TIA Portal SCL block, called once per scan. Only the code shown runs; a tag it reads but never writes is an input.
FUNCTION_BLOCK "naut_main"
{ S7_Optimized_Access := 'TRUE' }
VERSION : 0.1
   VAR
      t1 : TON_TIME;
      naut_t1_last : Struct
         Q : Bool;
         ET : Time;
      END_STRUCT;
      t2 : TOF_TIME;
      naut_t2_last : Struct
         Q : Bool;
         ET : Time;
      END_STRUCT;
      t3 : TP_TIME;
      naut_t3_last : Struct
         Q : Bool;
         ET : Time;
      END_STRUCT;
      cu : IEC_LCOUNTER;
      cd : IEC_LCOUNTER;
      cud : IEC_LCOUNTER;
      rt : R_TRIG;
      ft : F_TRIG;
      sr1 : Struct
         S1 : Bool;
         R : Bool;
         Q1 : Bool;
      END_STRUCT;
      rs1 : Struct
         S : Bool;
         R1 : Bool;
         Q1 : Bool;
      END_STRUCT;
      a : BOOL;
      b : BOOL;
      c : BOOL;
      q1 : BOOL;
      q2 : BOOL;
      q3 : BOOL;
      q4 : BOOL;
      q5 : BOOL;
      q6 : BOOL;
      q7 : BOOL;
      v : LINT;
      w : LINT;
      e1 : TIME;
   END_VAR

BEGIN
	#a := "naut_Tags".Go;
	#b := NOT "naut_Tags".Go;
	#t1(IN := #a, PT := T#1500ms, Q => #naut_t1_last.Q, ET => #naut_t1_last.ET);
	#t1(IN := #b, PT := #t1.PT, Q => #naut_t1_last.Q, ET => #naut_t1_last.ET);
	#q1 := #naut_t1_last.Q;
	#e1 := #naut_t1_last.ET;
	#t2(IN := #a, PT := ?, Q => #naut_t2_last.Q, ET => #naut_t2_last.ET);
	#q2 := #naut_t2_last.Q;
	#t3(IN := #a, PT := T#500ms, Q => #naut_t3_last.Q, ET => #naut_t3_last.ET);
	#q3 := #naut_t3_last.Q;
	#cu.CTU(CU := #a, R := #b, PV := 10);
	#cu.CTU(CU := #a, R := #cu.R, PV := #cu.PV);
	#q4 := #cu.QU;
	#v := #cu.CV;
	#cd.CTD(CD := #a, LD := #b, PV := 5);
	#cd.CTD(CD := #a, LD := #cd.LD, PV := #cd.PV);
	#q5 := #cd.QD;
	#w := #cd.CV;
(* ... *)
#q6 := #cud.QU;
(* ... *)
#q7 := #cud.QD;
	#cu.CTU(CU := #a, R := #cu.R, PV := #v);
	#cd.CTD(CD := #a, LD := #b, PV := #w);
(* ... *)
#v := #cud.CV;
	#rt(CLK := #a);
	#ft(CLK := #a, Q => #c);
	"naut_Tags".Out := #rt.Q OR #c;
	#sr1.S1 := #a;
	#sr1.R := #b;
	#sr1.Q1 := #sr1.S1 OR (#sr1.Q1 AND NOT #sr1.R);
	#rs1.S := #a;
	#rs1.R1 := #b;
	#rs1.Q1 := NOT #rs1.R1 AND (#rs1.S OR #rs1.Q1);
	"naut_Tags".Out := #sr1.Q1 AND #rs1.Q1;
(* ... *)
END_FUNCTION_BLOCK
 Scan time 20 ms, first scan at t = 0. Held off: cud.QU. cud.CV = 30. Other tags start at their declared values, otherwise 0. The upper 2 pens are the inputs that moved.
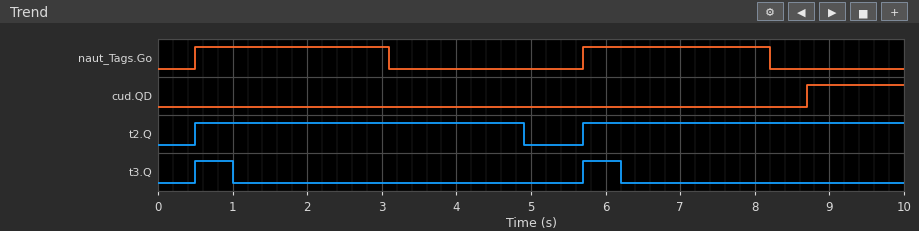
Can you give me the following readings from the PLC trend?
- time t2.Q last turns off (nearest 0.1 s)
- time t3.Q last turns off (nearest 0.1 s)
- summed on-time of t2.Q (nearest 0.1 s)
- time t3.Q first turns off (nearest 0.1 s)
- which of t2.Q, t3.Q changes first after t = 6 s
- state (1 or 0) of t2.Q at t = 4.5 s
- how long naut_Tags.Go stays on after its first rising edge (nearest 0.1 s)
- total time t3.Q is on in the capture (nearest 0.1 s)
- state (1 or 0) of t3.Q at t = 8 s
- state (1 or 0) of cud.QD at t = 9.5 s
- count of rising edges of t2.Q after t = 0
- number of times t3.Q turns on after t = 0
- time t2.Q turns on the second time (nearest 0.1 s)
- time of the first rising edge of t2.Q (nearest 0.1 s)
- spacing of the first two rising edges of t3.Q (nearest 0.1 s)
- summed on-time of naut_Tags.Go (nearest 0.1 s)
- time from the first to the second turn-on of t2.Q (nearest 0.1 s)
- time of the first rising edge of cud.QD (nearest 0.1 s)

4.9 s
6.2 s
8.7 s
1.0 s
t3.Q
1
2.6 s
1.0 s
0
1
2
2
5.7 s
0.5 s
5.2 s
5.1 s
5.2 s
8.7 s
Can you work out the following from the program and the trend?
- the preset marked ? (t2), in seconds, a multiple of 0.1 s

1.8 s
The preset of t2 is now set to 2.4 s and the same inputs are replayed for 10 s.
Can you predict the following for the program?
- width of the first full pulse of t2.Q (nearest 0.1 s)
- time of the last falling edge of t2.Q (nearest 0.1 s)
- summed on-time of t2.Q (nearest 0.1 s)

5.0 s
5.5 s
9.3 s
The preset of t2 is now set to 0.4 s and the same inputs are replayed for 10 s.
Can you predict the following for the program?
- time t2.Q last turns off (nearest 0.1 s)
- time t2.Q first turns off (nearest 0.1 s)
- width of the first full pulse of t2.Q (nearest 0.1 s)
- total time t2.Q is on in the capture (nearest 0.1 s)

8.6 s
3.5 s
3.0 s
5.9 s
